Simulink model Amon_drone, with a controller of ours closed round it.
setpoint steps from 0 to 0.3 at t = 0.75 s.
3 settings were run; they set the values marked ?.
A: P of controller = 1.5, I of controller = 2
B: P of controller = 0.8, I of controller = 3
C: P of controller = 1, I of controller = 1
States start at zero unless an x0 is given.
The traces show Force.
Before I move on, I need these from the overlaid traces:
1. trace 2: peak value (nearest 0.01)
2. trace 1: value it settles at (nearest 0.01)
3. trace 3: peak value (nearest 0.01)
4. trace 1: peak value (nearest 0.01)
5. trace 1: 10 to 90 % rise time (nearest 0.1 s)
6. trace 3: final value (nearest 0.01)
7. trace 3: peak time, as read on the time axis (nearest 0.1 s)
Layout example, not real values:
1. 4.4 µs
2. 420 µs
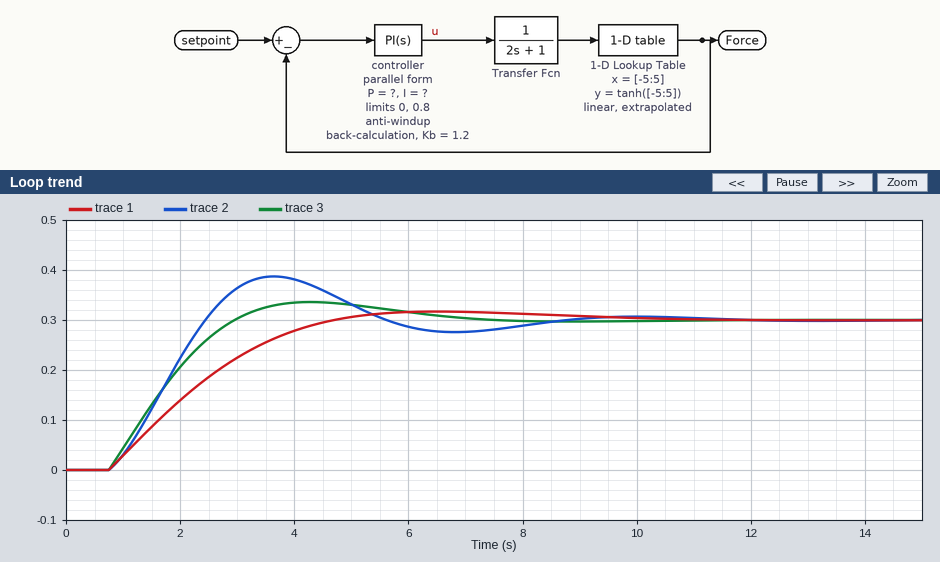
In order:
1. 0.39
2. 0.30
3. 0.34
4. 0.32
5. 2.8 s
6. 0.30
7. 4.3 s
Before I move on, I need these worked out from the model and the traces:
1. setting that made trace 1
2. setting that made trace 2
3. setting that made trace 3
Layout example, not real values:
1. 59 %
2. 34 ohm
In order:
1. C
2. B
3. A
